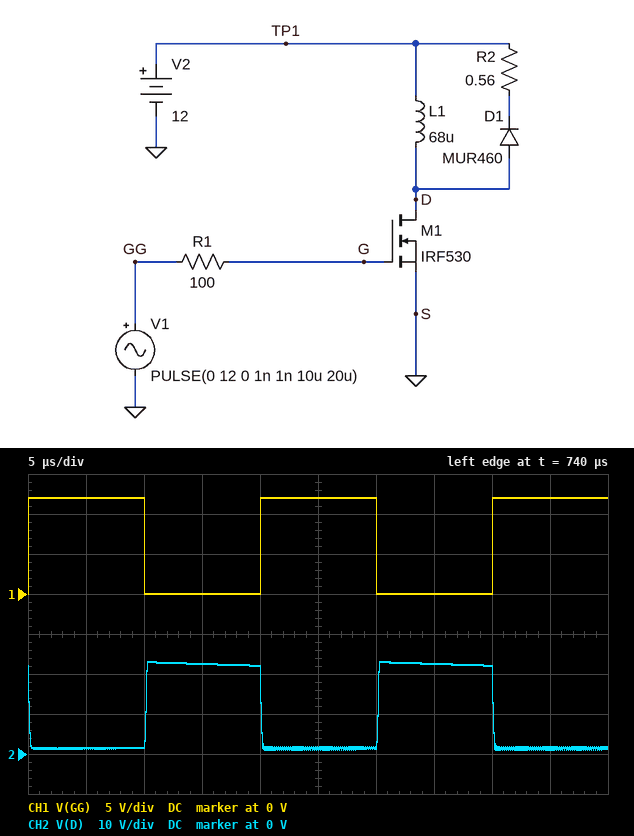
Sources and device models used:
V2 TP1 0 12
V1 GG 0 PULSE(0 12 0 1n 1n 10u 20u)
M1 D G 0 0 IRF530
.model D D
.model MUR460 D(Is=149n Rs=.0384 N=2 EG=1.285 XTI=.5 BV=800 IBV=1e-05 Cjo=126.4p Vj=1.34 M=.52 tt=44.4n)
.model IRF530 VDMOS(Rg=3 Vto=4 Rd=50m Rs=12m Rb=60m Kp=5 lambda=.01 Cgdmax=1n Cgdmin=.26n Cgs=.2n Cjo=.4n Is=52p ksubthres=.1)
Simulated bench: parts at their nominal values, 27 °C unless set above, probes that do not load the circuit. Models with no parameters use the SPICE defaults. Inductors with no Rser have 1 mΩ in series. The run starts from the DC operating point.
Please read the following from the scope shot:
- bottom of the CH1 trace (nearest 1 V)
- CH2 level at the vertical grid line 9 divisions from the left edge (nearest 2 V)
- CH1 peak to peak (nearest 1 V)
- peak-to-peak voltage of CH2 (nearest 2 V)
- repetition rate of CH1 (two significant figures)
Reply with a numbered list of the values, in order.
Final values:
1. 0 V
2. 2 V
3. 12 V
4. 22 V
5. 50 kHz
